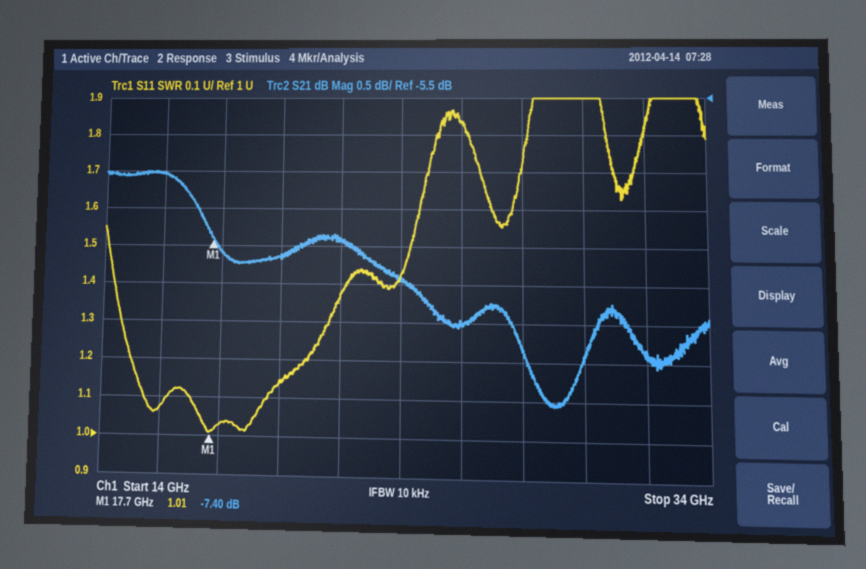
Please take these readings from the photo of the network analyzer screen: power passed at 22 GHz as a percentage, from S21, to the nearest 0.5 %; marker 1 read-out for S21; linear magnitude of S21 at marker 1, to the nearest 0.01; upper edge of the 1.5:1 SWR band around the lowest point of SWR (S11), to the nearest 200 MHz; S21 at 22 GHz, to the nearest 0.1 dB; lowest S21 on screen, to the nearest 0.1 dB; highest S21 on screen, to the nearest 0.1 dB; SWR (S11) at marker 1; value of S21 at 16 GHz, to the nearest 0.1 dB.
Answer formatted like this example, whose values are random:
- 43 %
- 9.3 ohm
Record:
- 18.0 %
- -7.40 dB
- 0.43
- 24.4 GHz
- -7.4 dB
- -9.6 dB
- -6.5 dB
- 1.01
- -6.5 dB
